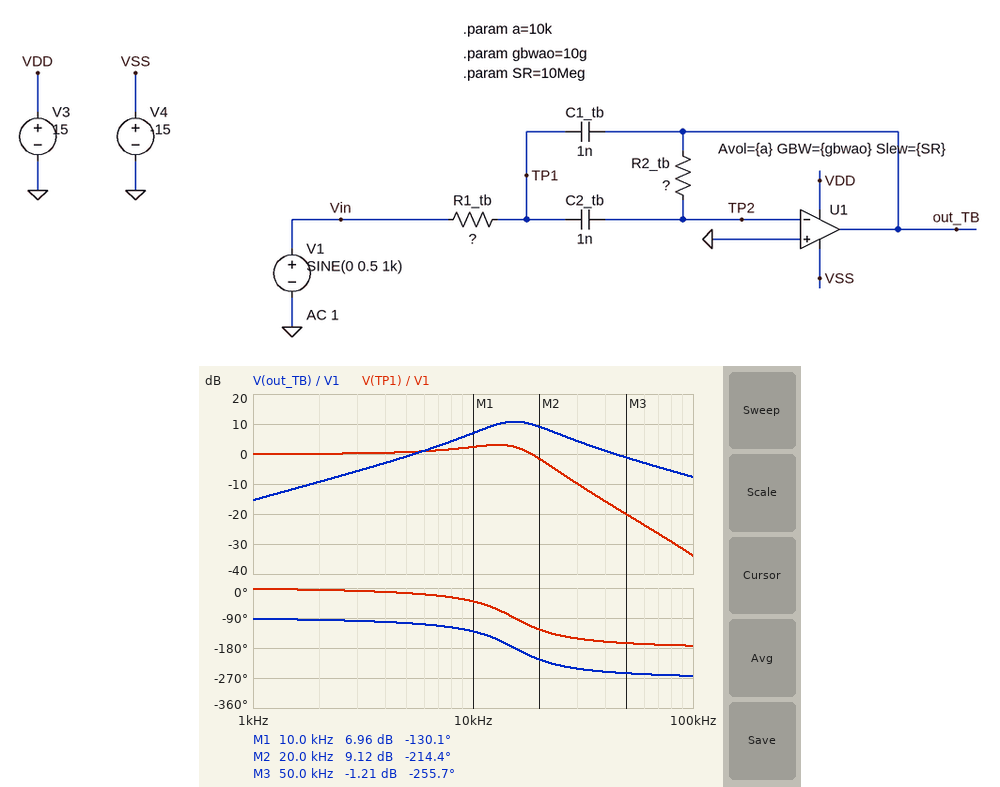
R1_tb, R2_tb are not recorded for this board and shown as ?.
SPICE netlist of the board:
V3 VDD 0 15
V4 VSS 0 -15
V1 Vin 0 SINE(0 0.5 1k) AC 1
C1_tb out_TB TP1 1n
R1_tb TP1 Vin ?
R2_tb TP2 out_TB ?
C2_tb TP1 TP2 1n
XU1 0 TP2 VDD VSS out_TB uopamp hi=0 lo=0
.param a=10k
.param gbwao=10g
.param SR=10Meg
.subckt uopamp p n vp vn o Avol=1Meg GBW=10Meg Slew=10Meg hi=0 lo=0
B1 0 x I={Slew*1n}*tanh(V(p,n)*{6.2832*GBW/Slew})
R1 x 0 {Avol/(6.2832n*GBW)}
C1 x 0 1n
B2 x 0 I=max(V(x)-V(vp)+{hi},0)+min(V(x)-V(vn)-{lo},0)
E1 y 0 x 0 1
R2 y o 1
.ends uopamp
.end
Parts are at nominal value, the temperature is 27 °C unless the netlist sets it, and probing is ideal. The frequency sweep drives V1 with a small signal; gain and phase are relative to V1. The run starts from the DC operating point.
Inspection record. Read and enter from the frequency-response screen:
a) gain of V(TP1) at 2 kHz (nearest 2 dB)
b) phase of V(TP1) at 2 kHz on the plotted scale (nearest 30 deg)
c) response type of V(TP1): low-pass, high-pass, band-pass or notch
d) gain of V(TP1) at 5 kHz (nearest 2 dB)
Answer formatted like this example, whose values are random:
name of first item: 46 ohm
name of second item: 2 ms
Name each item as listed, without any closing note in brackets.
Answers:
gain of V(TP1) at 2 kHz: 0 dB
phase of V(TP1) at 2 kHz on the plotted scale: 0 deg
response type of V(TP1): low-pass, high-pass, band-pass or notch: low-pass
gain of V(TP1) at 5 kHz: 0 dB
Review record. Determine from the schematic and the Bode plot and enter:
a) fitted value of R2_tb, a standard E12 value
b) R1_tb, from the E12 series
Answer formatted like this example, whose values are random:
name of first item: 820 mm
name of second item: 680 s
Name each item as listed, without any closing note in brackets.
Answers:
fitted value of R2_tb, a standard E12 value: 27 kΩ
R1_tb, from the E12 series: 3.9 kΩ
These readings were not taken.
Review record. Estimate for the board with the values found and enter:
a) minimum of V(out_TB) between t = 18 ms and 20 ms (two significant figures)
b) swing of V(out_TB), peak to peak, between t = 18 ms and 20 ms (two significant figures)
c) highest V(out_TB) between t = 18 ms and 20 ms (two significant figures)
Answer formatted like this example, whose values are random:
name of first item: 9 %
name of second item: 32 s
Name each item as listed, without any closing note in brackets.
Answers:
minimum of V(out_TB) between t = 18 ms and 20 ms: -85 mV
swing of V(out_TB), peak to peak, between t = 18 ms and 20 ms: 170 mV
highest V(out_TB) between t = 18 ms and 20 ms: 85 mV
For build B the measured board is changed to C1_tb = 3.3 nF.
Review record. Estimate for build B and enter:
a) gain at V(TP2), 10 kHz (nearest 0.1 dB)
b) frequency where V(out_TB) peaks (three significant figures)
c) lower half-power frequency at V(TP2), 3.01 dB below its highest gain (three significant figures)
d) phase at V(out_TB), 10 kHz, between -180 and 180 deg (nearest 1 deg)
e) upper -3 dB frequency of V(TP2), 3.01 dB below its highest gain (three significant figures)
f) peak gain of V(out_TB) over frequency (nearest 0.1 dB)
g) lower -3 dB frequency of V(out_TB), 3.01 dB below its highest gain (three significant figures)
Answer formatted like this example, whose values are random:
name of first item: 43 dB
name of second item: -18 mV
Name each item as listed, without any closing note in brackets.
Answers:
gain at V(TP2), 10 kHz: -56.4 dB
frequency where V(out_TB) peaks: 8.53 kHz
lower half-power frequency at V(TP2), 3.01 dB below its highest gain: 7.21 kHz
phase at V(out_TB), 10 kHz, between -180 and 180 deg: 160 deg
upper -3 dB frequency of V(TP2), 3.01 dB below its highest gain: 5.55 MHz
peak gain of V(out_TB) over frequency: 4.1 dB
lower -3 dB frequency of V(out_TB), 3.01 dB below its highest gain: 5.52 kHz
